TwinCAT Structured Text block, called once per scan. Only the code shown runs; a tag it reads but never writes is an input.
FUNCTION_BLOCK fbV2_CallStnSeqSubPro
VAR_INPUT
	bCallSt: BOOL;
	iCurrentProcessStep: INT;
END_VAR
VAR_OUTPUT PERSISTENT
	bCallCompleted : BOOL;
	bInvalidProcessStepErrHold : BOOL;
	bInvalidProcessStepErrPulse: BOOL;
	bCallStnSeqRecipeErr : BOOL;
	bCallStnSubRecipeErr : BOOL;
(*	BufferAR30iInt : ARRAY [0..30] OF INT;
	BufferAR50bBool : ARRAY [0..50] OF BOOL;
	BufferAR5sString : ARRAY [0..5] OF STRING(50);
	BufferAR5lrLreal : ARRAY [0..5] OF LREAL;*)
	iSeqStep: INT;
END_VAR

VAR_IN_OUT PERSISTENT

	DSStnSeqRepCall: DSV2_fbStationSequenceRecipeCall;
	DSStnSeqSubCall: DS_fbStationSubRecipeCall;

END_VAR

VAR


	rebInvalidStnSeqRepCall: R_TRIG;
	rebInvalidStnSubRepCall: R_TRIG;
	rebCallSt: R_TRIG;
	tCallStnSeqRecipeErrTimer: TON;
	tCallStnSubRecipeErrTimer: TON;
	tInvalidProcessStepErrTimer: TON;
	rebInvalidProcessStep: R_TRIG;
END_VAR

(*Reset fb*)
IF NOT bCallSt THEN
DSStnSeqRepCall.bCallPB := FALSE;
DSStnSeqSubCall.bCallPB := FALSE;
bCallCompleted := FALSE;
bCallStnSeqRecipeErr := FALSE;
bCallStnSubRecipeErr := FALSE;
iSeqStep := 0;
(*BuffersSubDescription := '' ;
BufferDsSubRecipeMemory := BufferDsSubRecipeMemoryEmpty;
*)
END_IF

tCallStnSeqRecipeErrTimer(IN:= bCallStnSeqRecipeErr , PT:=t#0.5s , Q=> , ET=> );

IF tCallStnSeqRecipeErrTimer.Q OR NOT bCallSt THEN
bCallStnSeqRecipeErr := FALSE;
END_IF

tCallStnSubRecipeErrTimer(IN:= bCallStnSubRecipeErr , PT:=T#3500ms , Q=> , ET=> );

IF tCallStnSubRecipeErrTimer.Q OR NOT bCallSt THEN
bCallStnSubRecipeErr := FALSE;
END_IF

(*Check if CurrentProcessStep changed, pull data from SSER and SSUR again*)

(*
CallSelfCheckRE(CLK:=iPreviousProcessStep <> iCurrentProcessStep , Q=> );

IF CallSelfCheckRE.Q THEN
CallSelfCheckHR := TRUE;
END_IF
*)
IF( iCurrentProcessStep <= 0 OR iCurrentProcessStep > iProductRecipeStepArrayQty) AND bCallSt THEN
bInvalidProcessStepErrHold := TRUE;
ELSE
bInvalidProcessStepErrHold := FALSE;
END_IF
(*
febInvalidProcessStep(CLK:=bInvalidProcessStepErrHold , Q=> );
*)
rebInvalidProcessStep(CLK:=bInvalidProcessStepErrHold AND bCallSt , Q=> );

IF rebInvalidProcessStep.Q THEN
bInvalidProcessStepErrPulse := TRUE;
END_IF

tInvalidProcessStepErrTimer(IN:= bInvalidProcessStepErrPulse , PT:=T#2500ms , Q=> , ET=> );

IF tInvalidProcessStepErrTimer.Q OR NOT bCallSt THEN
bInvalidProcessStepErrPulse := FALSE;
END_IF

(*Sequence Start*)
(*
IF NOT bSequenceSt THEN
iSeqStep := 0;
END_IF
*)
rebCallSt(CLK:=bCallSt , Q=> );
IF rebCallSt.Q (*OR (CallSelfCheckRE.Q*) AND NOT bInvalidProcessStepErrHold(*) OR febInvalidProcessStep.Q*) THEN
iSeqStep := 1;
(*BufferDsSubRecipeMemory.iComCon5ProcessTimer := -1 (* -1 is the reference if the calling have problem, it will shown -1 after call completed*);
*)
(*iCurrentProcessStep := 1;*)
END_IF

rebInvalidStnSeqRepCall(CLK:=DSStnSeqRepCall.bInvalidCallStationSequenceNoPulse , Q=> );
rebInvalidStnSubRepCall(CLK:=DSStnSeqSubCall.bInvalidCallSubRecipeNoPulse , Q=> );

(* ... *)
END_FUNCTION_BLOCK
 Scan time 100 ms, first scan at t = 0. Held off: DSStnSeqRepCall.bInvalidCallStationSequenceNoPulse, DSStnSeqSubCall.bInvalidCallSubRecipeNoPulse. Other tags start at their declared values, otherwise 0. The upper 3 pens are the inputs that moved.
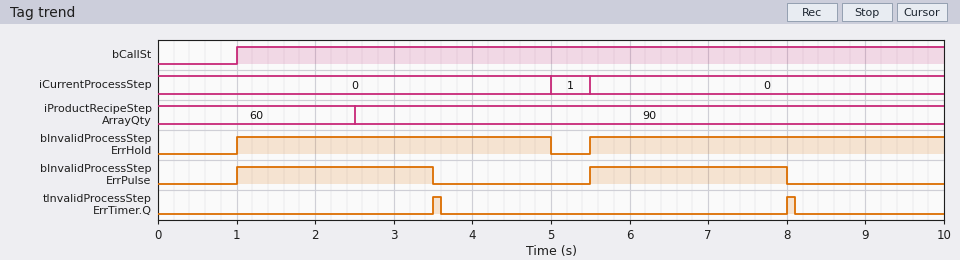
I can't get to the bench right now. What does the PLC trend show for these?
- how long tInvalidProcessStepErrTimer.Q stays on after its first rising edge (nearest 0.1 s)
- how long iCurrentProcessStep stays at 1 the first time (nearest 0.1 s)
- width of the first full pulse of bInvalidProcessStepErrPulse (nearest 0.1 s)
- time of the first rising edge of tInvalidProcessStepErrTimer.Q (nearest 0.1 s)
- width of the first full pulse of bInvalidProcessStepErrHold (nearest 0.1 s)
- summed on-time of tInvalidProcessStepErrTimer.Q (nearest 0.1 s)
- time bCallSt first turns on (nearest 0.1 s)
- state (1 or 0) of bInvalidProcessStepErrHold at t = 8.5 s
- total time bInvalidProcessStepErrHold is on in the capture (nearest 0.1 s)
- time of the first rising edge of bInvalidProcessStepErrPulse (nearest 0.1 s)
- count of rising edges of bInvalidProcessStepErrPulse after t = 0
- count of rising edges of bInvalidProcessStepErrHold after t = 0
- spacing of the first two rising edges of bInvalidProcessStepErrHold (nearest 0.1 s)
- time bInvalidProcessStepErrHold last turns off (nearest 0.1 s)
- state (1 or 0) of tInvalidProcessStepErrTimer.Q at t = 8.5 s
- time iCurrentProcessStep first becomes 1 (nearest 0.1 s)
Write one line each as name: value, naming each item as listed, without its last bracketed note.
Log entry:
how long tInvalidProcessStepErrTimer.Q stays on after its first rising edge: 0.1 s
how long iCurrentProcessStep stays at 1 the first time: 0.5 s
width of the first full pulse of bInvalidProcessStepErrPulse: 2.5 s
time of the first rising edge of tInvalidProcessStepErrTimer.Q: 3.5 s
width of the first full pulse of bInvalidProcessStepErrHold: 4.0 s
summed on-time of tInvalidProcessStepErrTimer.Q: 0.2 s
time bCallSt first turns on: 1.0 s
state (1 or 0) of bInvalidProcessStepErrHold at t = 8.5 s: 1
total time bInvalidProcessStepErrHold is on in the capture: 8.5 s
time of the first rising edge of bInvalidProcessStepErrPulse: 1.0 s
count of rising edges of bInvalidProcessStepErrPulse after t = 0: 2
count of rising edges of bInvalidProcessStepErrHold after t = 0: 2
spacing of the first two rising edges of bInvalidProcessStepErrHold: 4.5 s
time bInvalidProcessStepErrHold last turns off: 5.0 s
state (1 or 0) of tInvalidProcessStepErrTimer.Q at t = 8.5 s: 0
time iCurrentProcessStep first becomes 1: 5.0 s
